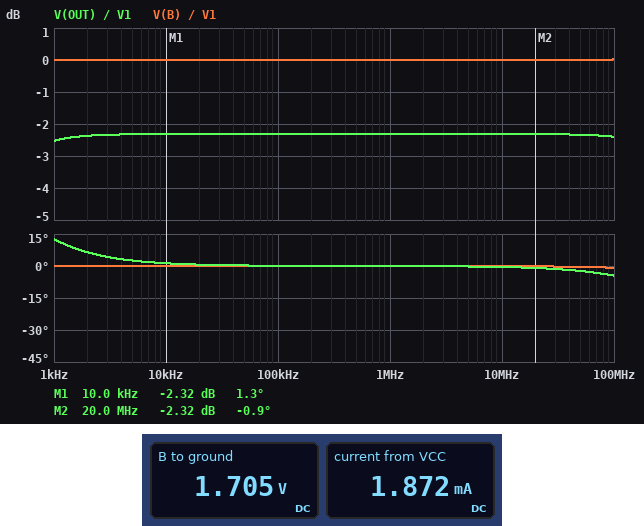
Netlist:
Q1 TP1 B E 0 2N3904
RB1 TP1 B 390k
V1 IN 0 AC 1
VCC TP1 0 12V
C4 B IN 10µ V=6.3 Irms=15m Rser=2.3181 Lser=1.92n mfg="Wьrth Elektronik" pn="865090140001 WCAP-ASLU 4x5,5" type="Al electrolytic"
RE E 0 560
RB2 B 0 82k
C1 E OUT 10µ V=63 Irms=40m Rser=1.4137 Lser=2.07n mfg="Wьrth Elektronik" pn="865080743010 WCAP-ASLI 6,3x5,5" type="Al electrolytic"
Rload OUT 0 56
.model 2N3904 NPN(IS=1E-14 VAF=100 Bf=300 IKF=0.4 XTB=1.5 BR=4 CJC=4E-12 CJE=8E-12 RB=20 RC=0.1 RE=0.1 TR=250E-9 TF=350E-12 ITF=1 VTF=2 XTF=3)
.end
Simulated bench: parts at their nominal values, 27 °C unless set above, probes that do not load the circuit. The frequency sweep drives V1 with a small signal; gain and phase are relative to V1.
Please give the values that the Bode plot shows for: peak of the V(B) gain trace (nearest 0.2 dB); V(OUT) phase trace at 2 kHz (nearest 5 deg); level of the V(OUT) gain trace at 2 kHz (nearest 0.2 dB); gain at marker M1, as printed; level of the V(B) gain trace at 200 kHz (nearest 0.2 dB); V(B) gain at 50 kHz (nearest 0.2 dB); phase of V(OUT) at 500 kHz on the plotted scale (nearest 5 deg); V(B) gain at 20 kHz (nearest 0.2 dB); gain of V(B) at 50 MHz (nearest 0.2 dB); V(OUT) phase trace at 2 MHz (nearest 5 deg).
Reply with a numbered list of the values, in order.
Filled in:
1. 0 dB
2. 5 deg
3. -2.4 dB
4. -2.32 dB
5. 0 dB
6. 0 dB
7. 0 deg
8. 0 dB
9. 0 dB
10. 0 deg
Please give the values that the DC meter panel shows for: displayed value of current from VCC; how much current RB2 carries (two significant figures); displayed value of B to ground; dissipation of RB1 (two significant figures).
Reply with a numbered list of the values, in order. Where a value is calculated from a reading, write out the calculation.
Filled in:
1. 1.872 mA
2. (1.705 V) / 82 kΩ = 21 µA
3. 1.705 V
4. (12 V - 1.705 V)^2 / 390 kΩ = 270 µW
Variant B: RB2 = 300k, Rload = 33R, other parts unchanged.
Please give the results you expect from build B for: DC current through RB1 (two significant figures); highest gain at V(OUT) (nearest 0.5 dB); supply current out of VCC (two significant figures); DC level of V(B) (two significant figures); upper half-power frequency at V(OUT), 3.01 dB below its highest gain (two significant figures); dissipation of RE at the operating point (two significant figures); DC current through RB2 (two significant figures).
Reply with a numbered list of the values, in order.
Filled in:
1. 23 µA
2. -2.0 dB
3. 4.2 mA
4. 3.0 V
5. 1.0 GHz
6. 9.8 mW
7. 10 µA
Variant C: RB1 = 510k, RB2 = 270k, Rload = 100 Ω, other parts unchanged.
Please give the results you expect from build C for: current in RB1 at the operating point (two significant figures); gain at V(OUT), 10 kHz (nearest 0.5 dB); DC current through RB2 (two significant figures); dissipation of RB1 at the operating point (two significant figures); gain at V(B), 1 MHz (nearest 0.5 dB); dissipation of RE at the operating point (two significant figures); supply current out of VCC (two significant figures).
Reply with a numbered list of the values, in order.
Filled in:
1. 19 µA
2. -1.0 dB
3. 9.1 µA
4. 180 µW
5. 0 dB
6. 5.6 mW
7. 3.2 mA
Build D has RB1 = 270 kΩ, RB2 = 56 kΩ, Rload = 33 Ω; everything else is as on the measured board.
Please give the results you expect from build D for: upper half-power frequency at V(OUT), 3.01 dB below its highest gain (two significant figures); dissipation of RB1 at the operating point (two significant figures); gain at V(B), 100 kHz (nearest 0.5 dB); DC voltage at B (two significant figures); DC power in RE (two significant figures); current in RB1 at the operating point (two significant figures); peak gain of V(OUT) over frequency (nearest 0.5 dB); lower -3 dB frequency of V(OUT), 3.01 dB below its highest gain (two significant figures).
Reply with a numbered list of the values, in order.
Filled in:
1. 3.7 GHz
2. 390 µW
3. 0 dB
4. 1.8 V
5. 2.2 mW
6. 38 µA
7. -3.5 dB
8. 340 Hz
